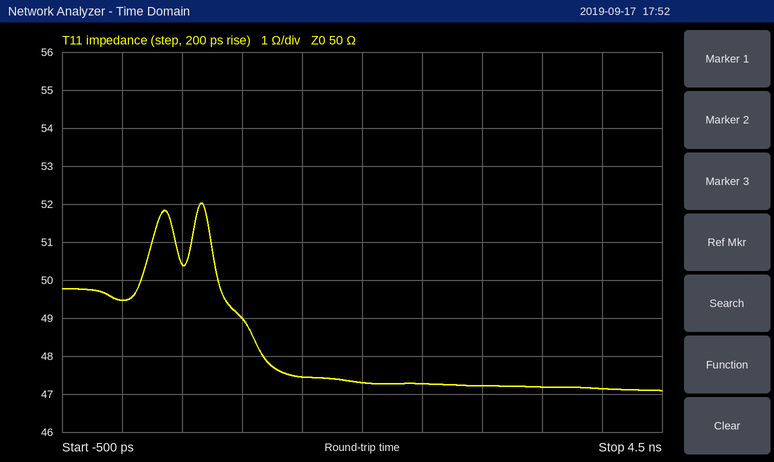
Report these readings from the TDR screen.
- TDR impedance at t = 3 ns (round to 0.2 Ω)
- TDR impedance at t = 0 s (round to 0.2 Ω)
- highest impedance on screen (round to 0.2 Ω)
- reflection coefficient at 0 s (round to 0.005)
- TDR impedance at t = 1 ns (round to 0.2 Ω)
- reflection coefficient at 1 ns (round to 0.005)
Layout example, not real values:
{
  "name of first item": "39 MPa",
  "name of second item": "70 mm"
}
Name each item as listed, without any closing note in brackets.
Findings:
{
  "TDR impedance at t = 3 ns": "47.2 Ω",
  "TDR impedance at t = 0 s": "49.4 Ω",
  "highest impedance on screen": "52.0 Ω",
  "reflection coefficient at 0 s": "-0.005",
  "TDR impedance at t = 1 ns": "49.0 Ω",
  "reflection coefficient at 1 ns": "-0.010"
}
